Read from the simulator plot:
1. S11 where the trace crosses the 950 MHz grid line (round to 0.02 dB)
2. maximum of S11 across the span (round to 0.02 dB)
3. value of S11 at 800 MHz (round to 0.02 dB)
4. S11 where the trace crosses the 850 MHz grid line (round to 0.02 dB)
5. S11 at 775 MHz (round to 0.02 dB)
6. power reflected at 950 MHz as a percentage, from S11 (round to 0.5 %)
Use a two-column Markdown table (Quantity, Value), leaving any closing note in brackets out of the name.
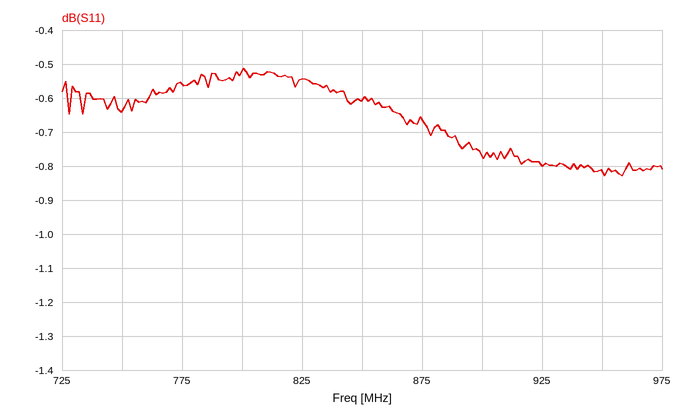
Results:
| Quantity | Value |
|---|---|
| S11 where the trace crosses the 950 MHz grid line | -0.82 dB |
| maximum of S11 across the span | -0.52 dB |
| value of S11 at 800 MHz | -0.52 dB |
| S11 where the trace crosses the 850 MHz grid line | -0.60 dB |
| S11 at 775 MHz | -0.56 dB |
| power reflected at 950 MHz as a percentage, from S11 | 83.0 % |
